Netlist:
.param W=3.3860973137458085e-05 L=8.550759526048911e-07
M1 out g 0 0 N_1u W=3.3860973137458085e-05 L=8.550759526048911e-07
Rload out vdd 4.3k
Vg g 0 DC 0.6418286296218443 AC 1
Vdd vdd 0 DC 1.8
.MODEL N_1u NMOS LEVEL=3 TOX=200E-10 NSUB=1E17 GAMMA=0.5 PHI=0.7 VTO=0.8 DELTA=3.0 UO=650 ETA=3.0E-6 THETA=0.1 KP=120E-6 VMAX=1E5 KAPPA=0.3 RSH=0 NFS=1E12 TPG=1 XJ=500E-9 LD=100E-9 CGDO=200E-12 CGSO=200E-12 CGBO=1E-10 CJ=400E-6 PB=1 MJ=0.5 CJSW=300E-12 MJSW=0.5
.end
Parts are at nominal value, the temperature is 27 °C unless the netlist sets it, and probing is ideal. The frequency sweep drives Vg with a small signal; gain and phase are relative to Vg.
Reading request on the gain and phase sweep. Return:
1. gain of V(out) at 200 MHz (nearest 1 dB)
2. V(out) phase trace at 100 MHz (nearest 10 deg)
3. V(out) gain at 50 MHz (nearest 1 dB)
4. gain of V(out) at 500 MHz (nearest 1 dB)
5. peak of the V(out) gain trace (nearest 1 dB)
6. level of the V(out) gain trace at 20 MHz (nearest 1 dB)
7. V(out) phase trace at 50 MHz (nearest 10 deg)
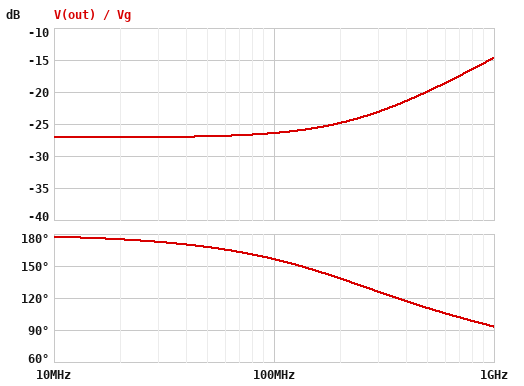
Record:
-25 dB
160 deg
-27 dB
-20 dB
-15 dB
-27 dB
170 deg
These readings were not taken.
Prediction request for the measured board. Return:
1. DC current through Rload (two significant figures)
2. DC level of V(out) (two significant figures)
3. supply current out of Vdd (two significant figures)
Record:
580 nA
1.8 V
580 nA
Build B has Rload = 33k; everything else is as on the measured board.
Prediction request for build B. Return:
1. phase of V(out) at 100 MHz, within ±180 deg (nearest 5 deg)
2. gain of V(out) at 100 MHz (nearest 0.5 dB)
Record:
150 deg
-9.0 dB
